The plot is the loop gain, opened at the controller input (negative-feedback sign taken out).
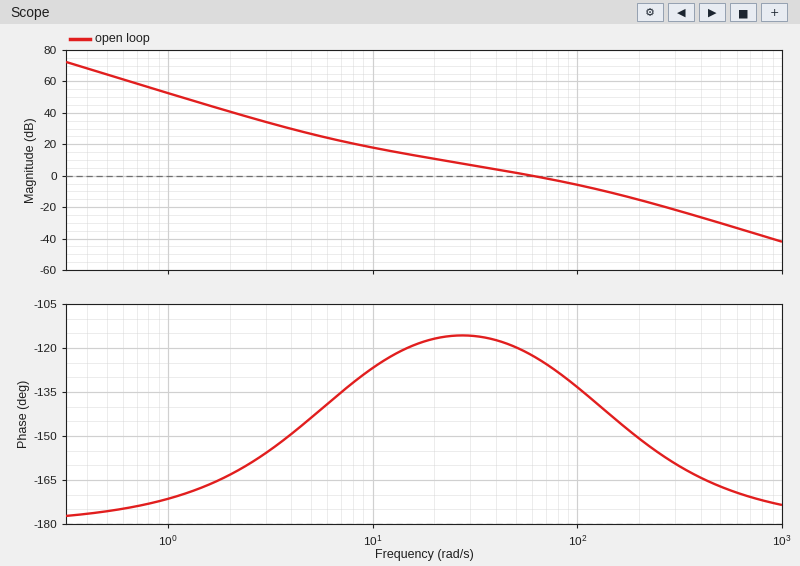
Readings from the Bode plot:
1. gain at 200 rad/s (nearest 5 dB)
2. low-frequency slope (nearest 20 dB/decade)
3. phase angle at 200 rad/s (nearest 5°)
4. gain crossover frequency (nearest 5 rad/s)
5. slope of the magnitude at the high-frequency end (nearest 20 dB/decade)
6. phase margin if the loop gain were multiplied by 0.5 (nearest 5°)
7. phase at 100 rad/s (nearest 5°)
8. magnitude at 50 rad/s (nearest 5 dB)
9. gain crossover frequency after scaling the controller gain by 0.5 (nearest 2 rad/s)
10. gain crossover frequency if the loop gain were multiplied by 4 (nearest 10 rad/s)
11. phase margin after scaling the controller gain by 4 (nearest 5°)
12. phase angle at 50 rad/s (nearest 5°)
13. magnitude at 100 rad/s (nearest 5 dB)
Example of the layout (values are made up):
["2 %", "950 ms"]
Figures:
["-15 dB", "-40 dB/decade", "-150°", "60 rad/s", "-40 dB/decade", "65°", "-135°", "0 dB", "32 rad/s", "160 rad/s", "35°", "-120°", "-5 dB"]
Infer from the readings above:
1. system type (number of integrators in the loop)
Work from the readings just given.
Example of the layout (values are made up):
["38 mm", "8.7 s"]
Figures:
["2"]
